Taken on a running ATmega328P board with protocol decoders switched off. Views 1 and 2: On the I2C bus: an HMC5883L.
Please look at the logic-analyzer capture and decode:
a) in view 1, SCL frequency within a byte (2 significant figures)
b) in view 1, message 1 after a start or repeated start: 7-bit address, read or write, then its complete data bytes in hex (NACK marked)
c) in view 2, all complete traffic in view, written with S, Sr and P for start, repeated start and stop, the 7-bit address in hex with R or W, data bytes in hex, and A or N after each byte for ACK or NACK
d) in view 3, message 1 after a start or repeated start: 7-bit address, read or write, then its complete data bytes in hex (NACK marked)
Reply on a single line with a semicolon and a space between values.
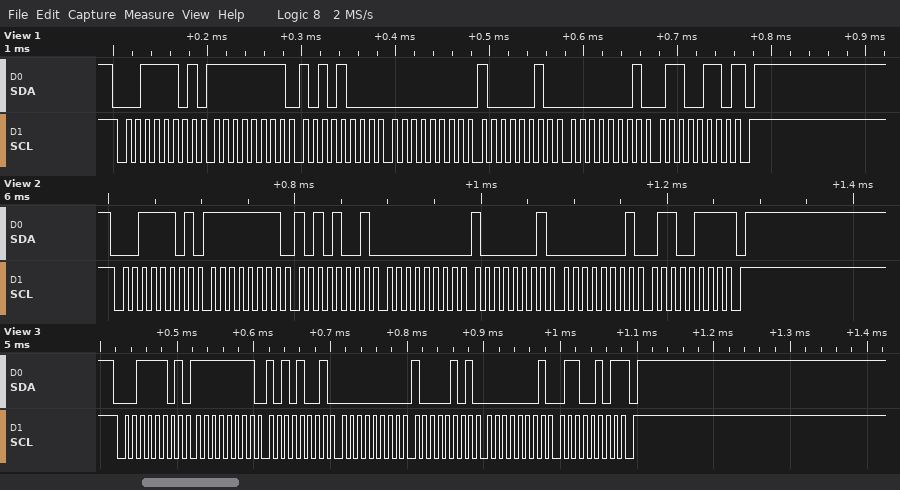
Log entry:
100 kHz; 0x1E read: FF A8 00 82 01 66 NACK; S 1ER A FF A A9 A 00 A 81 A 01 A 67 N P; 0x1E read: FF A9 00 85 01 65 NACK
